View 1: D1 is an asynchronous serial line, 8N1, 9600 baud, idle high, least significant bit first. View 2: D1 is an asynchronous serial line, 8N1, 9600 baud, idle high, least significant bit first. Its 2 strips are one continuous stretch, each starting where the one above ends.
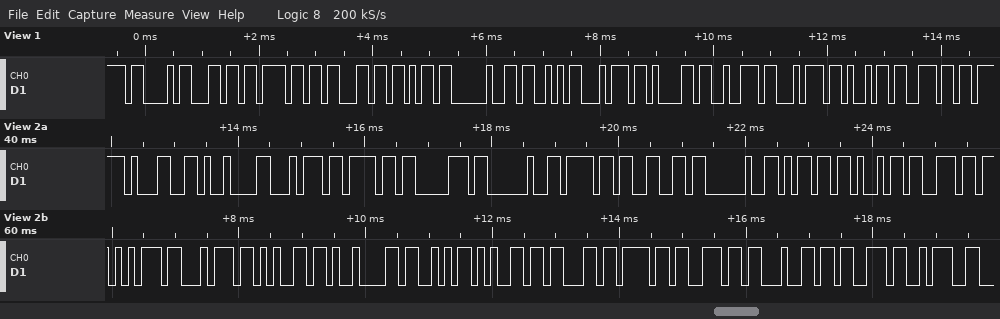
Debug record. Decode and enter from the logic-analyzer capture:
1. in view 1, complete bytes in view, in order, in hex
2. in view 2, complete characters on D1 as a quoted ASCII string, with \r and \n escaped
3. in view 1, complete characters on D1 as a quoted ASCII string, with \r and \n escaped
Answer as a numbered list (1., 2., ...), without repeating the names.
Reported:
1. 43 6C 6F 63 6B 20 53 74 61 72 74 69 6E
2. "1\ttop of minute\tSeconds:"
3. "Clock Startin"
